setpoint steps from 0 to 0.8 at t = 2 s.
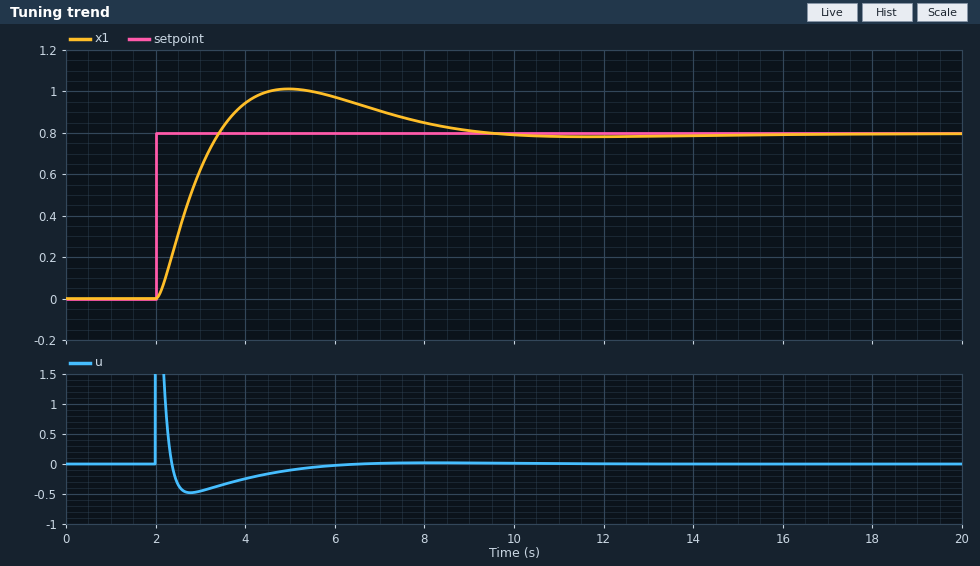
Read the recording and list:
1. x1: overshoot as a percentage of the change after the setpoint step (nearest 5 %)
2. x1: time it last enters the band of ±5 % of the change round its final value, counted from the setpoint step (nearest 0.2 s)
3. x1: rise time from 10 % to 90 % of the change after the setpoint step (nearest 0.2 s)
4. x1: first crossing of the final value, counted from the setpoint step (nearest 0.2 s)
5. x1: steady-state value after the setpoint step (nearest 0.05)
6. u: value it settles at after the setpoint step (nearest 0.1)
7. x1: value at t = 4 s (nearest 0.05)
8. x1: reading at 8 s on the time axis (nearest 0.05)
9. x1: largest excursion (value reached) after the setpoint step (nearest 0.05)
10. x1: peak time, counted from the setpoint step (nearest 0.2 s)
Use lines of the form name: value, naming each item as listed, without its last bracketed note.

x1: overshoot as a percentage of the change after the setpoint step: 25 %
x1: time it last enters the band of ±5 % of the change round its final value, counted from the setpoint step: 6.2 s
x1: rise time from 10 % to 90 % of the change after the setpoint step: 1.0 s
x1: first crossing of the final value, counted from the setpoint step: 1.4 s
x1: steady-state value after the setpoint step: 0.80
u: value it settles at after the setpoint step: 0.0
x1: value at t = 4 s: 0.95
x1: reading at 8 s on the time axis: 0.85
x1: largest excursion (value reached) after the setpoint step: 1.00
x1: peak time, counted from the setpoint step: 3.0 s
